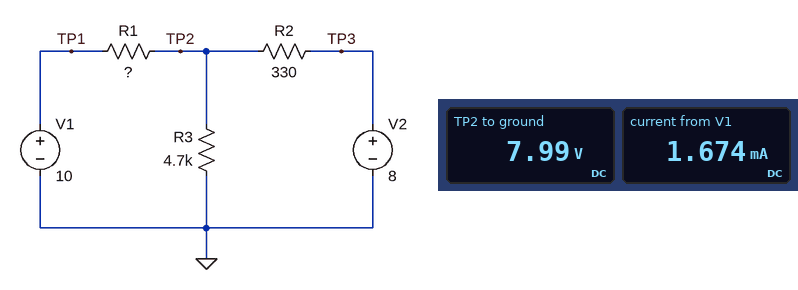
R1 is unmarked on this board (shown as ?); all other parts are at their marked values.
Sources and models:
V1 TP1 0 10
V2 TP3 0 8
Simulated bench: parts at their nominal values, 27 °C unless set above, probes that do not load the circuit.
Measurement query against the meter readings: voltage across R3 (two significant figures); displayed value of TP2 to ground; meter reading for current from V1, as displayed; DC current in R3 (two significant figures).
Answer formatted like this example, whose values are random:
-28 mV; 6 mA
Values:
8.0 V; 7.99 V; 1.674 mA; 1.7 mA
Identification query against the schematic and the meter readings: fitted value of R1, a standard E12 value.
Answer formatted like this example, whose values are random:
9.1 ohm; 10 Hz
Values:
1.2 kΩ
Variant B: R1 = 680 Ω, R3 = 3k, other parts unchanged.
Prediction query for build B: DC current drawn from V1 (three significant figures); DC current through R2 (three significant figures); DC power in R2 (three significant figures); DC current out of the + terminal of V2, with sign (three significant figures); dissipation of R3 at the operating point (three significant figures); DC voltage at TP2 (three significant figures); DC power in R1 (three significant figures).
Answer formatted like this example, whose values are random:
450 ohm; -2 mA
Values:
2.86 mA; 172 µA; 9.77 µW; -172 µA; 21.6 mW; 8.06 V; 5.55 mW
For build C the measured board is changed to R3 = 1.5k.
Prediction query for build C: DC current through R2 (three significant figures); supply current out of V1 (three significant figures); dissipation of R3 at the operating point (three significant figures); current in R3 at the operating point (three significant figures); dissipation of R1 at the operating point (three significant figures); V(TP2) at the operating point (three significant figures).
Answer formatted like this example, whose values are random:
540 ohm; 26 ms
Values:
2.45 mA; 2.34 mA; 34.5 mW; 4.79 mA; 6.58 mW; 7.19 V
